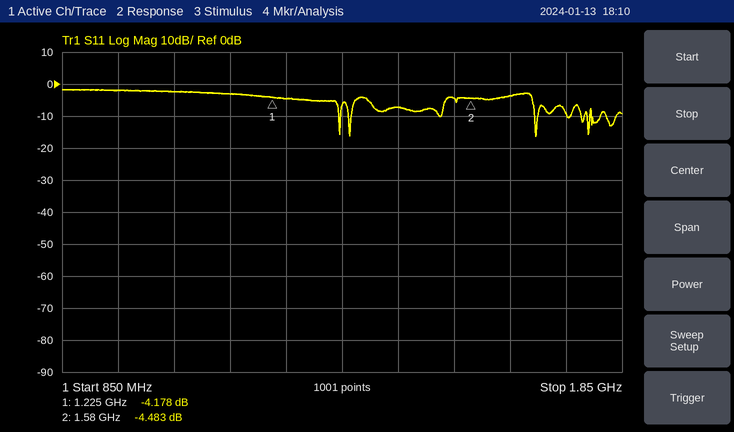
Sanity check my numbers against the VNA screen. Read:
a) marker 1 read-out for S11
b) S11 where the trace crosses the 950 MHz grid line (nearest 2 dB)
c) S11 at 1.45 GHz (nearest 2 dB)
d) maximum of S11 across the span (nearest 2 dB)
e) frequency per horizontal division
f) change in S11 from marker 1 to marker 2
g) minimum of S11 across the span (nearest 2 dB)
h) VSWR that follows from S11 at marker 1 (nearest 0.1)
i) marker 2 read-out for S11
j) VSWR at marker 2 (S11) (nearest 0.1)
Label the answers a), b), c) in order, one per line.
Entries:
a) -4.178 dB
b) -2 dB
c) -8 dB
d) -2 dB
e) 100 MHz
f) -0.305 dB
g) -16 dB
h) 4.2
i) -4.483 dB
j) 4.0
